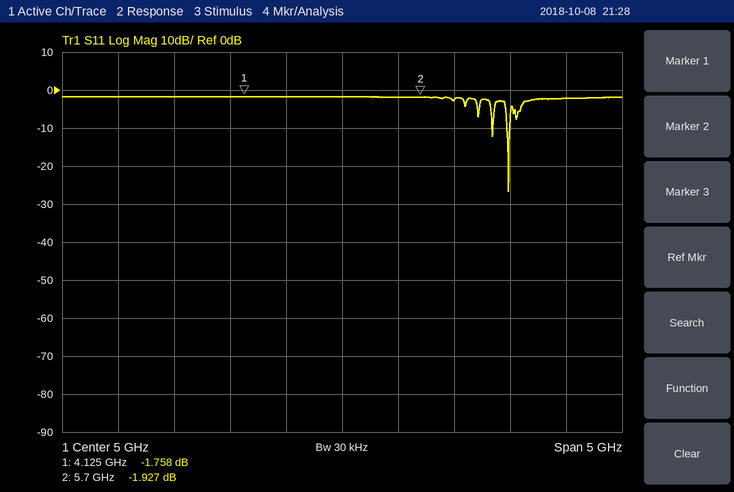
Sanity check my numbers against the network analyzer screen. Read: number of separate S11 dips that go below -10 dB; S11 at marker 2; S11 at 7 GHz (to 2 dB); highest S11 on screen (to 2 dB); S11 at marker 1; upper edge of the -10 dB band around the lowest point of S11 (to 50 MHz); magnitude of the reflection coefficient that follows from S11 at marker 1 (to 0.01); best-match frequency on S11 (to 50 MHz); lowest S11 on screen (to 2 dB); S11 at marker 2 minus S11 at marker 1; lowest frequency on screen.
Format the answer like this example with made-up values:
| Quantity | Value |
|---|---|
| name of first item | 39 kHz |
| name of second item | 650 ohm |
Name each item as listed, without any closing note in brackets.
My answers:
| Quantity | Value |
|---|---|
| number of separate S11 dips that go below -10 dB | 2 |
| S11 at marker 2 | -1.927 dB |
| S11 at 7 GHz | -2 dB |
| highest S11 on screen | -2 dB |
| S11 at marker 1 | -1.758 dB |
| upper edge of the -10 dB band around the lowest point of S11 | 6.50 GHz |
| magnitude of the reflection coefficient that follows from S11 at marker 1 | 0.82 |
| best-match frequency on S11 | 6.50 GHz |
| lowest S11 on screen | -26 dB |
| S11 at marker 2 minus S11 at marker 1 | -0.169 dB |
| lowest frequency on screen | 2.5 GHz |
